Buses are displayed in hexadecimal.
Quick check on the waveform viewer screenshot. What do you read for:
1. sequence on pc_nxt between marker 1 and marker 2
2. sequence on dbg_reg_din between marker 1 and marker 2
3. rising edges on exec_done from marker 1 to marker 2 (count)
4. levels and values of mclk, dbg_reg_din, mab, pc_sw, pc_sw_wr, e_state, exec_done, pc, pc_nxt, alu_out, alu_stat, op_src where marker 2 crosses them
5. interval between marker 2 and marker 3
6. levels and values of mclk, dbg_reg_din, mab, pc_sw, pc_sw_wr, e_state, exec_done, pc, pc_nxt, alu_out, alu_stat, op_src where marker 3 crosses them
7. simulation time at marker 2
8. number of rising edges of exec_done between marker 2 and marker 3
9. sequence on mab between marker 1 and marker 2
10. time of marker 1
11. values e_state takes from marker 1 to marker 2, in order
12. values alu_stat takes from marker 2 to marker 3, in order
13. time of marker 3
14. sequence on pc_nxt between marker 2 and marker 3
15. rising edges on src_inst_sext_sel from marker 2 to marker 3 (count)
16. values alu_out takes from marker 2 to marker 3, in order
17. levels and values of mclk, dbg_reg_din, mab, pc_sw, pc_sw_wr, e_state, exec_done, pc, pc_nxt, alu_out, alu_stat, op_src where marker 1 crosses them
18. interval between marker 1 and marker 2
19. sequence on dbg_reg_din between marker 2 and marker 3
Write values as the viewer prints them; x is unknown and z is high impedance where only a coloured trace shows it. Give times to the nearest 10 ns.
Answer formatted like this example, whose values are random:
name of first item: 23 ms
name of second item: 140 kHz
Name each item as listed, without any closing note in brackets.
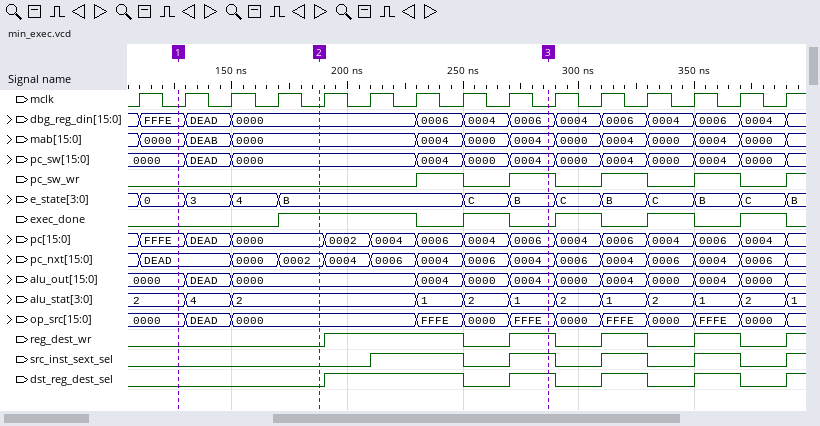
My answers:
sequence on pc_nxt between marker 1 and marker 2: DEAD, 0000, 0002
sequence on dbg_reg_din between marker 1 and marker 2: FFFE, DEAD, 0000
rising edges on exec_done from marker 1 to marker 2: 1
levels and values of mclk, dbg_reg_din, mab, pc_sw, pc_sw_wr, e_state, exec_done, pc, pc_nxt, alu_out, alu_stat, op_src where marker 2 crosses them: mclk=0, dbg_reg_din=0000, mab=0000, pc_sw=0000, pc_sw_wr=0, e_state=B, exec_done=1, pc=0000, pc_nxt=0002, alu_out=0000, alu_stat=2, op_src=0000
interval between marker 2 and marker 3: 100 ns
levels and values of mclk, dbg_reg_din, mab, pc_sw, pc_sw_wr, e_state, exec_done, pc, pc_nxt, alu_out, alu_stat, op_src where marker 3 crosses them: mclk=0, dbg_reg_din=0006, mab=0004, pc_sw=0004, pc_sw_wr=1, e_state=B, exec_done=0, pc=0006, pc_nxt=0004, alu_out=0004, alu_stat=1, op_src=FFFE
simulation time at marker 2: 190 ns
number of rising edges of exec_done between marker 2 and marker 3: 1
sequence on mab between marker 1 and marker 2: 0000, DEAB, 0000
time of marker 1: 130 ns
values e_state takes from marker 1 to marker 2, in order: 0, 3, 4, B
values alu_stat takes from marker 2 to marker 3, in order: 2, 1, 2, 1
time of marker 3: 290 ns
sequence on pc_nxt between marker 2 and marker 3: 0002, 0004, 0006, 0004, 0006, 0004
rising edges on src_inst_sext_sel from marker 2 to marker 3: 2
values alu_out takes from marker 2 to marker 3, in order: 0000, 0004, 0000, 0004
levels and values of mclk, dbg_reg_din, mab, pc_sw, pc_sw_wr, e_state, exec_done, pc, pc_nxt, alu_out, alu_stat, op_src where marker 1 crosses them: mclk=0, dbg_reg_din=FFFE, mab=0000, pc_sw=0000, pc_sw_wr=0, e_state=0, exec_done=0, pc=FFFE, pc_nxt=DEAD, alu_out=0000, alu_stat=2, op_src=0000
interval between marker 1 and marker 2: 60 ns
sequence on dbg_reg_din between marker 2 and marker 3: 0000, 0006, 0004, 0006
